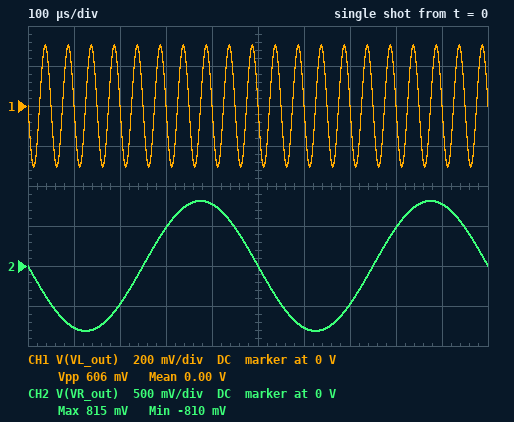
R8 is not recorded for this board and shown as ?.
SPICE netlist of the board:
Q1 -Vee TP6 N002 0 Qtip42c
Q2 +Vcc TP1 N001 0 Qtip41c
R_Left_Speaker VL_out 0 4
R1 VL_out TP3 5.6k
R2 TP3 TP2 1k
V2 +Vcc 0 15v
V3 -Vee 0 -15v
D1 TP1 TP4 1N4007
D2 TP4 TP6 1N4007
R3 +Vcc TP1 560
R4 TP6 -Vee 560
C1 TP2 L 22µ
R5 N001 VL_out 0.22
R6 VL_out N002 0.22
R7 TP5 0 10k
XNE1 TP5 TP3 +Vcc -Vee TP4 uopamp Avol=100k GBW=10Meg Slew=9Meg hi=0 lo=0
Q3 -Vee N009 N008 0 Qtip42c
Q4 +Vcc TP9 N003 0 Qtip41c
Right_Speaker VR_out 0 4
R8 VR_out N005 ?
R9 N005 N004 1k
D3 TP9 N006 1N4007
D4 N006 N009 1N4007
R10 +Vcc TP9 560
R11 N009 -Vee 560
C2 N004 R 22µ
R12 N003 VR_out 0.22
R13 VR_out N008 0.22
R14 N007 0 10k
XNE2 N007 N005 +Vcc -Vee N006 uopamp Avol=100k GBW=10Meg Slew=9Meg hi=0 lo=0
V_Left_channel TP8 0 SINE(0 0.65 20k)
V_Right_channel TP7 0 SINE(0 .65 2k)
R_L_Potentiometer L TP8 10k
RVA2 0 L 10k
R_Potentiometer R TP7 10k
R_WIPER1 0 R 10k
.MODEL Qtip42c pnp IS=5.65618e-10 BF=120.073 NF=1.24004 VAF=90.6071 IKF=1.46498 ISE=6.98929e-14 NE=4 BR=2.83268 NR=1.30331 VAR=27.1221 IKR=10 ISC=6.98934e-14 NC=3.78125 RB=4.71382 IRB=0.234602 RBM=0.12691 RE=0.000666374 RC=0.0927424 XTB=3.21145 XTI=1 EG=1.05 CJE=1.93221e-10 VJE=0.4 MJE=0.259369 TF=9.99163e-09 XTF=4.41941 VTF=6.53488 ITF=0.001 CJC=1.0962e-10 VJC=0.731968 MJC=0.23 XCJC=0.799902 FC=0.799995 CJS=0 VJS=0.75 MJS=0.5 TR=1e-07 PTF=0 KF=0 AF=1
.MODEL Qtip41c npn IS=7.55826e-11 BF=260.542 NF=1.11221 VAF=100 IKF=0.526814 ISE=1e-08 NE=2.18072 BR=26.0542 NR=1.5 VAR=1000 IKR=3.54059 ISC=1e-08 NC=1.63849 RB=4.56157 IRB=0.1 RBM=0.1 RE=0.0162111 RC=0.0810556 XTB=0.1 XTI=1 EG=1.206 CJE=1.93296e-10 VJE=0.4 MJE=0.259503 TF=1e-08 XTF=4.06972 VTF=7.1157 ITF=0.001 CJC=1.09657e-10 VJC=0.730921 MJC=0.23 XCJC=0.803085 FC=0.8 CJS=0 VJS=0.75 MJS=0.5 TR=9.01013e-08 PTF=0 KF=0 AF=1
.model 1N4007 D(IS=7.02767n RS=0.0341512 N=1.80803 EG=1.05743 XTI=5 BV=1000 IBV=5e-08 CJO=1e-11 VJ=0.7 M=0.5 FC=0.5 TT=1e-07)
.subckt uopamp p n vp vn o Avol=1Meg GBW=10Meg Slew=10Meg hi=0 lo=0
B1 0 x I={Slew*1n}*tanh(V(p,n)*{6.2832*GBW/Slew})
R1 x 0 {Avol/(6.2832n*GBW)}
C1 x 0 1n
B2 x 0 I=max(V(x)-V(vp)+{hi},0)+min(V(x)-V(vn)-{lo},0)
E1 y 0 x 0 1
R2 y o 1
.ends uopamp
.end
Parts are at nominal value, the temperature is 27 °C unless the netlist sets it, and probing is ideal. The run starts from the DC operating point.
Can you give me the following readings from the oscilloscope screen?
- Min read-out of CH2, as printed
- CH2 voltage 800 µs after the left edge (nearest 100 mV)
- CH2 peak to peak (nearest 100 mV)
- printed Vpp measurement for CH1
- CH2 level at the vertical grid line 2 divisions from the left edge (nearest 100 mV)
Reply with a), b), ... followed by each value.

a) -810 mV
b) 500 mV
c) 1.6 V
d) 606 mV
e) -500 mV
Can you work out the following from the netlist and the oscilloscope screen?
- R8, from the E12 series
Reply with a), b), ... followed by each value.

a) 15 kΩ
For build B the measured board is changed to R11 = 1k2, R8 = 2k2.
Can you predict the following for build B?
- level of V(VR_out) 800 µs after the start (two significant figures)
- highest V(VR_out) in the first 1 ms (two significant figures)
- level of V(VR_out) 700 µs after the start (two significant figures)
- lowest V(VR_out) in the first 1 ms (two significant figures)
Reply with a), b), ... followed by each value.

a) 70 mV
b) 120 mV
c) -70 mV
d) -120 mV
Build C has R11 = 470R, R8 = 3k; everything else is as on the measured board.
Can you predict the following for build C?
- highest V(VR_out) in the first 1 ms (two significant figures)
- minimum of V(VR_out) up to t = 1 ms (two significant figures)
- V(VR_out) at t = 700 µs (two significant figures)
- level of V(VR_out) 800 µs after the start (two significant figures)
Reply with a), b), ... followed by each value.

a) 160 mV
b) -160 mV
c) -95 mV
d) 96 mV
